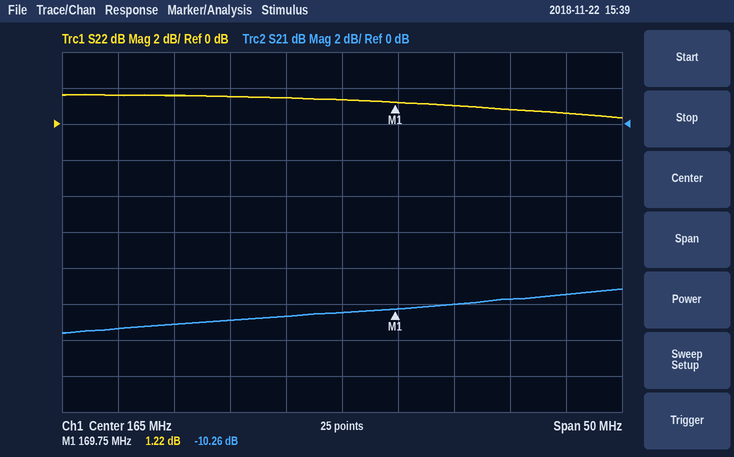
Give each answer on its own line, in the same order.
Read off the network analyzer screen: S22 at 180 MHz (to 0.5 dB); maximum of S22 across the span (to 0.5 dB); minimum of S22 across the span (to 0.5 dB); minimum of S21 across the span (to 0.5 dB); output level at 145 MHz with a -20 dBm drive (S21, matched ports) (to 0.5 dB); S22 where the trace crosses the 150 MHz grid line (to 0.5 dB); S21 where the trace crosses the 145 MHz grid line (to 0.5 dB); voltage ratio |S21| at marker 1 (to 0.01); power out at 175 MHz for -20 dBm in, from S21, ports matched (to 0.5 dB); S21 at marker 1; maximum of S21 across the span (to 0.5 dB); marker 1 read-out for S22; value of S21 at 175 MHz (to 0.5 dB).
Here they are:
1.0 dB
1.5 dB
0.5 dB
-11.5 dB
-31.5 dBm
1.5 dB
-11.5 dB
0.31
-30.0 dBm
-10.26 dB
-9.0 dB
1.22 dB
-10.0 dB
